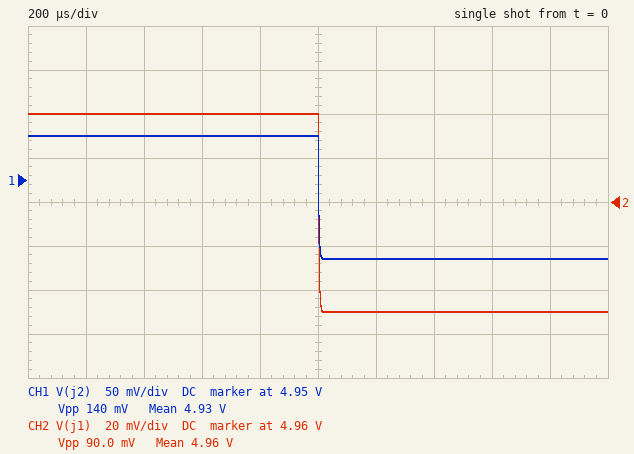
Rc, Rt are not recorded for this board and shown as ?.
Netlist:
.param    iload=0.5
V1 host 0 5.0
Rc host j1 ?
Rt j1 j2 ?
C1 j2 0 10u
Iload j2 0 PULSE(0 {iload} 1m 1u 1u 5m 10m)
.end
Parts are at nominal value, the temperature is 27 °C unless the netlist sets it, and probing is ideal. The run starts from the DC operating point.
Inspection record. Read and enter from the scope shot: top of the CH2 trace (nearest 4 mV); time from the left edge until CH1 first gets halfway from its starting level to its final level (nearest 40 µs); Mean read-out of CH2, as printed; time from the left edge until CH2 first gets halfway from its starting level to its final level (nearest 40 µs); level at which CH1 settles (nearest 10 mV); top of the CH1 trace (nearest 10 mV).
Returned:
5.000 V
1.00 ms
4.96 V
1.00 ms
4.86 V
5.00 V
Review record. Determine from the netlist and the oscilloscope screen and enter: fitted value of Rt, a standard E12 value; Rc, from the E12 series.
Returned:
0.1 Ω
0.18 Ω
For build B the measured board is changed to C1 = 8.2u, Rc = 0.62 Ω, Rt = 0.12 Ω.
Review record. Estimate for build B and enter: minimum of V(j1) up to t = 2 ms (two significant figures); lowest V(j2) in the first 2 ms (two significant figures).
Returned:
4.7 V
4.6 V
